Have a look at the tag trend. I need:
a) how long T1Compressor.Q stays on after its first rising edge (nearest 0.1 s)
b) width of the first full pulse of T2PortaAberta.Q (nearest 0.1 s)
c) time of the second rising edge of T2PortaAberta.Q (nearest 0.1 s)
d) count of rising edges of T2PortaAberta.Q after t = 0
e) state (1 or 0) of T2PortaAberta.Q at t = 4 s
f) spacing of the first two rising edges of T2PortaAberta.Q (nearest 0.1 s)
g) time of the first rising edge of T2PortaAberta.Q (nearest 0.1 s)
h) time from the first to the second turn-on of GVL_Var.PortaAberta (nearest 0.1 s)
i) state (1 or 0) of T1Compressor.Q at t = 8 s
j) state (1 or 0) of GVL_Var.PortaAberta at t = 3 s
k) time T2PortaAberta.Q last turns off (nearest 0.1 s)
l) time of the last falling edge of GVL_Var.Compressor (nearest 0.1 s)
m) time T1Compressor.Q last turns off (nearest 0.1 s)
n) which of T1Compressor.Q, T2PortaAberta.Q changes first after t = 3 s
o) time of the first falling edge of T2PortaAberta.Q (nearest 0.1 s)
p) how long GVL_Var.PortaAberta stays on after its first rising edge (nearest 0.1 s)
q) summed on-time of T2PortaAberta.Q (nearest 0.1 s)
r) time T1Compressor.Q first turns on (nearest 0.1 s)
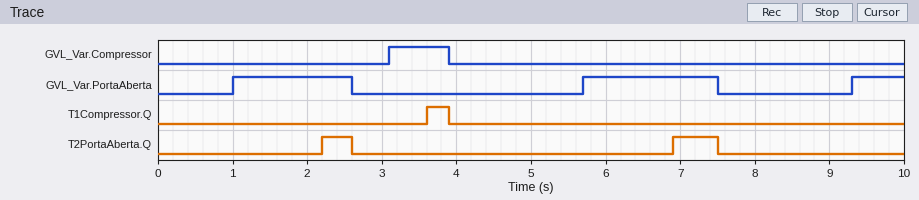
0.3 s
0.4 s
6.9 s
2
0
4.7 s
2.2 s
4.7 s
0
0
7.5 s
3.9 s
3.9 s
T1Compressor.Q
2.6 s
1.6 s
1.0 s
3.6 s
